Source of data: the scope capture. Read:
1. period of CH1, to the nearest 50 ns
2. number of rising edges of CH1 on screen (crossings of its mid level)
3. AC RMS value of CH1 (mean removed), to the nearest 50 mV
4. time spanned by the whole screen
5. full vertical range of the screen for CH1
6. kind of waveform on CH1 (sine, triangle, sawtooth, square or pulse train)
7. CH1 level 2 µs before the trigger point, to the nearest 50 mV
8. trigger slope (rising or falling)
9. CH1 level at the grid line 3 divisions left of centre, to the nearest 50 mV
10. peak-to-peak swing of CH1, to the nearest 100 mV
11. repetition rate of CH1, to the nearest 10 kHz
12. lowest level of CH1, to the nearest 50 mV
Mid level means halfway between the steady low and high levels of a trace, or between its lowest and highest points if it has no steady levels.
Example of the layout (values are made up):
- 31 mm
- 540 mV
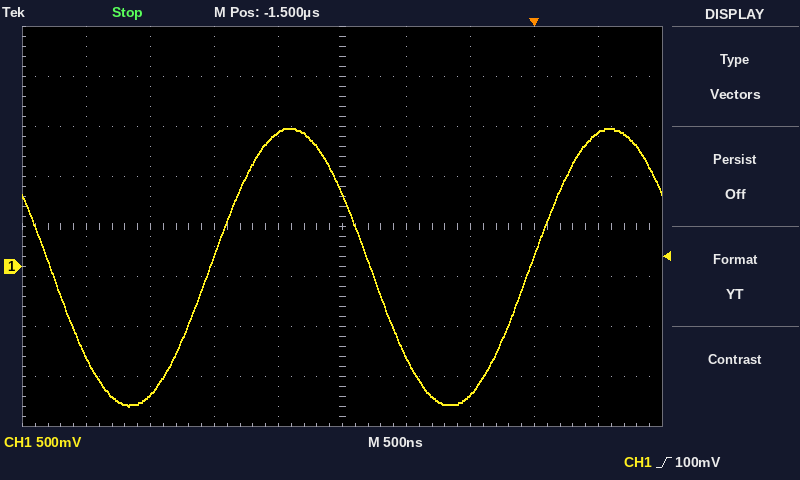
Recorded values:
- 2.50 µs
- 2
- 1.00 V
- 5 µs
- 4 V
- sine
- 1.35 V
- rising
- -1.30 V
- 2.80 V
- 400 kHz
- -1.40 V
